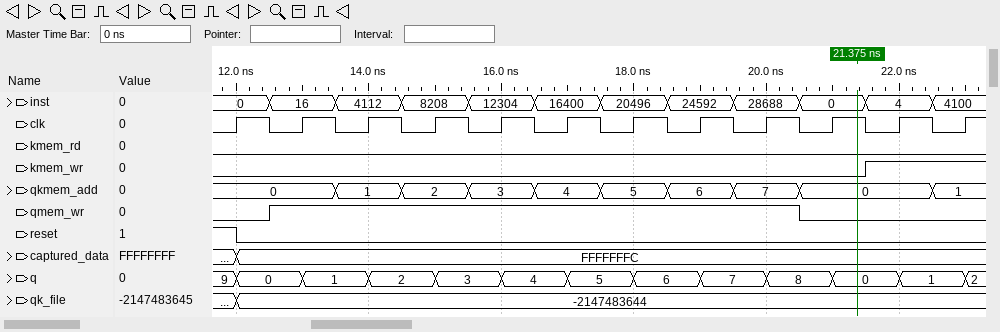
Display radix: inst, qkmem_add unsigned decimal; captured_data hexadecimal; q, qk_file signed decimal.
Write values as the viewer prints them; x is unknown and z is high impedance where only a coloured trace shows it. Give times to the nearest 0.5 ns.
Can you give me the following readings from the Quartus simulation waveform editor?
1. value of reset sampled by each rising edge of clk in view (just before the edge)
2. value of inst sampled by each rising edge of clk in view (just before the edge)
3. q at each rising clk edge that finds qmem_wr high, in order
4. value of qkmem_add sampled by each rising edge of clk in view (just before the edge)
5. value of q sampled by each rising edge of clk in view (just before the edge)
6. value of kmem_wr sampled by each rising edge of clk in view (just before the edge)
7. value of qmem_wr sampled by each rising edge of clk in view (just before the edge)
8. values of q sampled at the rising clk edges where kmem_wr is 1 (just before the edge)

1 0 0 0 0 0 0 0 0 0 0 0
0, 16, 4112, 8208, 12304, 16400, 20496, 24592, 28688, 0, 4, 4100
0, 1, 2, 3, 4, 5, 6, 7
0, 0, 1, 2, 3, 4, 5, 6, 7, 0, 0, 1
9, 0, 1, 2, 3, 4, 5, 6, 7, 8, 0, 1
0 0 0 0 0 0 0 0 0 0 1 1
0 1 1 1 1 1 1 1 1 0 0 0
0, 1
